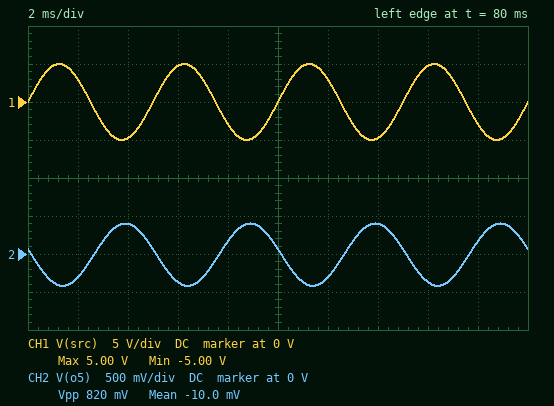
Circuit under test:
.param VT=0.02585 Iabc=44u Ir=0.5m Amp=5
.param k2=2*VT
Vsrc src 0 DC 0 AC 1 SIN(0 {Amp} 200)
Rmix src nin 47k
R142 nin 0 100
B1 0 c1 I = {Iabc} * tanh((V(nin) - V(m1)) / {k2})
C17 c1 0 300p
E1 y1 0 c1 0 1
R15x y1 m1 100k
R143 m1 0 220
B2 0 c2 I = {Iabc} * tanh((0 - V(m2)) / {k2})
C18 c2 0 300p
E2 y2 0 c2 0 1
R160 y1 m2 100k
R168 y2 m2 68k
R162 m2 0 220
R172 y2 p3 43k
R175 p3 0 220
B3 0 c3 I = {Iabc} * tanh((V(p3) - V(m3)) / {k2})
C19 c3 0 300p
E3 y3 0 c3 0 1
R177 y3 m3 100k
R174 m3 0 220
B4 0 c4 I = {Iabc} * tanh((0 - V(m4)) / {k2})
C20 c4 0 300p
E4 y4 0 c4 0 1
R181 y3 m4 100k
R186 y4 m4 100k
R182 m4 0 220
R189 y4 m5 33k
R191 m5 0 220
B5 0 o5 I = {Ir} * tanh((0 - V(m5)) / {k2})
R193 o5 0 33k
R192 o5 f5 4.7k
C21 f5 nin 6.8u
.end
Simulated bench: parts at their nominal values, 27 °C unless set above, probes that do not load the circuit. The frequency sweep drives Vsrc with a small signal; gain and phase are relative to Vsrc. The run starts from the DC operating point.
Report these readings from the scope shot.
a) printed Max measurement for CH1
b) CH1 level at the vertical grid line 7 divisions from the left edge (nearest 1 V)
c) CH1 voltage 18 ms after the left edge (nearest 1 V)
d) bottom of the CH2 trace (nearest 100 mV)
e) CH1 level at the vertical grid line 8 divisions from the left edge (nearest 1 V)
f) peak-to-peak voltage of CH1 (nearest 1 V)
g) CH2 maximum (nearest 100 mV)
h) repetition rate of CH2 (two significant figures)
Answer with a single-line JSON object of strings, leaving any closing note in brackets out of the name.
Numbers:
{"printed Max measurement for CH1": "5.00 V", "CH1 level at the vertical grid line 7 divisions from the left edge": "-5 V", "CH1 voltage 18 ms after the left edge": "-3 V", "bottom of the CH2 trace": "-400 mV", "CH1 level at the vertical grid line 8 divisions from the left edge": "5 V", "peak-to-peak voltage of CH1": "10 V", "CH2 maximum": "400 mV", "repetition rate of CH2": "200 Hz"}
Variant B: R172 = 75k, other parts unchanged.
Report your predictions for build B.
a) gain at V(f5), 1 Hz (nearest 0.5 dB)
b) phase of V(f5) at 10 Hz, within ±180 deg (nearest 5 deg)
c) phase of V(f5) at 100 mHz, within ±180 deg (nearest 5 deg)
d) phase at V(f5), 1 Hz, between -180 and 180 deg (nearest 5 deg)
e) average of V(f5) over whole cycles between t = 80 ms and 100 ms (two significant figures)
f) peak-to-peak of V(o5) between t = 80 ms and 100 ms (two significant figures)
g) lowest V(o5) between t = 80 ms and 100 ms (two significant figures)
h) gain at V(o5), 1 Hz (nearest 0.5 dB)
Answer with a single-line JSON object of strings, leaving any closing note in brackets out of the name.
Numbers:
{"gain at V(f5), 1 Hz": "-9.5 dB", "phase of V(f5) at 10 Hz, within ±180 deg": "90 deg", "phase of V(f5) at 100 mHz, within ±180 deg": "150 deg", "phase at V(f5), 1 Hz, between -180 and 180 deg": "100 deg", "average of V(f5) over whole cycles between t = 80 ms and 100 ms": "-7.8 mV", "peak-to-peak of V(o5) between t = 80 ms and 100 ms": "720 mV", "lowest V(o5) between t = 80 ms and 100 ms": "-370 mV", "gain at V(o5), 1 Hz": "-9.0 dB"}
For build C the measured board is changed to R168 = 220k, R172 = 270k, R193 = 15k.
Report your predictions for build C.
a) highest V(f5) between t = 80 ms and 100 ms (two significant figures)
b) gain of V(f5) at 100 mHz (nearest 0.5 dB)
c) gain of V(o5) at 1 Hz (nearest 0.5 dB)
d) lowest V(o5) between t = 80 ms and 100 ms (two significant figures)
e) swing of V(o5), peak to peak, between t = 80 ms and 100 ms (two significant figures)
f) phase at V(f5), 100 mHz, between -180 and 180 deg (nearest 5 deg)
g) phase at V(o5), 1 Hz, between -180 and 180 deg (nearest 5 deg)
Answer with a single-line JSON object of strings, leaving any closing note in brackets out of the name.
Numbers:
{"highest V(f5) between t = 80 ms and 100 ms": "6.6 mV", "gain of V(f5) at 100 mHz": "-2.5 dB", "gain of V(o5) at 1 Hz": "-10.5 dB", "lowest V(o5) between t = 80 ms and 100 ms": "-350 mV", "swing of V(o5), peak to peak, between t = 80 ms and 100 ms": "680 mV", "phase at V(f5), 100 mHz, between -180 and 180 deg": "165 deg", "phase at V(o5), 1 Hz, between -180 and 180 deg": "125 deg"}
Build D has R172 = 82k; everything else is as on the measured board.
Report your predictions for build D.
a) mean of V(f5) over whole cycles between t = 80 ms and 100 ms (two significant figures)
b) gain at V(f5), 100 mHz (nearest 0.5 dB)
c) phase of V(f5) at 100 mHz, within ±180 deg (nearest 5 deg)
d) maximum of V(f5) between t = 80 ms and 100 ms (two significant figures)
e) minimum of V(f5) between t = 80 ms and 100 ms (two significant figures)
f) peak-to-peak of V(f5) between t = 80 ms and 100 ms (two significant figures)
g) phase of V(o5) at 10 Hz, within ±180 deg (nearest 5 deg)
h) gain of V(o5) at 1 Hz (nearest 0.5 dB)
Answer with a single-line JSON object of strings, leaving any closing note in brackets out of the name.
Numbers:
{"mean of V(f5) over whole cycles between t = 80 ms and 100 ms": "-7.5 mV", "gain at V(f5), 100 mHz": "3.5 dB", "phase of V(f5) at 100 mHz, within ±180 deg": "155 deg", "maximum of V(f5) between t = 80 ms and 100 ms": "4.2 mV", "minimum of V(f5) between t = 80 ms and 100 ms": "-19 mV", "peak-to-peak of V(f5) between t = 80 ms and 100 ms": "23 mV", "phase of V(o5) at 10 Hz, within ±180 deg": "155 deg", "gain of V(o5) at 1 Hz": "-9.5 dB"}
